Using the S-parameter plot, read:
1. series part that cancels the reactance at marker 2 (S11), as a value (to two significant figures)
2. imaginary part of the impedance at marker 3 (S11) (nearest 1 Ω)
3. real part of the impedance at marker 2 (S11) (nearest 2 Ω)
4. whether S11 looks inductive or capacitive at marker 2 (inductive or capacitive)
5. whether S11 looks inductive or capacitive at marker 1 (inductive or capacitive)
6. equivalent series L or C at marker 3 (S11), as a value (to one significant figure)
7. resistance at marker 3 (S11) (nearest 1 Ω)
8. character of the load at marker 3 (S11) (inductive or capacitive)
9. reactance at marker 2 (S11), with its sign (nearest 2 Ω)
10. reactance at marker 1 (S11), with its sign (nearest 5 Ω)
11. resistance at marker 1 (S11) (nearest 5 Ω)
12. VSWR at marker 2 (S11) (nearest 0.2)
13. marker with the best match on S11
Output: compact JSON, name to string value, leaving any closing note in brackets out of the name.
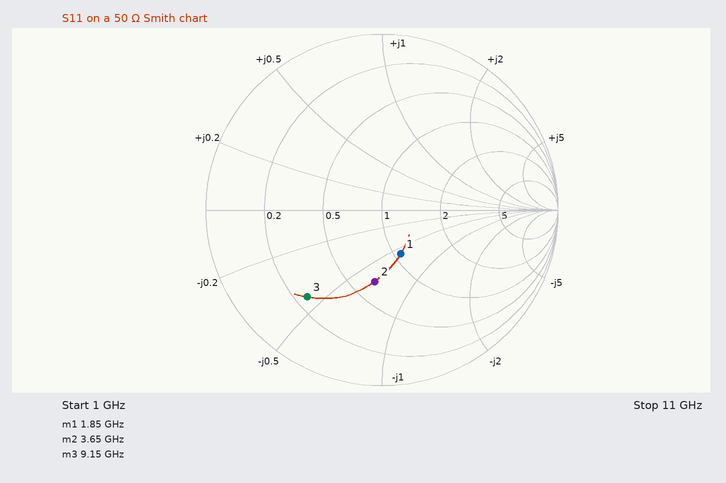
{"series part that cancels the reactance at marker 2 (S11), as a value": "1.4 nH", "imaginary part of the impedance at marker 3 (S11)": "-22 Ω", "real part of the impedance at marker 2 (S11)": "34 Ω", "whether S11 looks inductive or capacitive at marker 2": "capacitive", "whether S11 looks inductive or capacitive at marker 1": "capacitive", "equivalent series L or C at marker 3 (S11), as a value": "800 fF", "resistance at marker 3 (S11)": "13 Ω", "character of the load at marker 3 (S11)": "capacitive", "reactance at marker 2 (S11), with its sign": "-32 Ω", "reactance at marker 1 (S11), with its sign": "-30 Ω", "resistance at marker 1 (S11)": "55 Ω", "VSWR at marker 2 (S11)": "2.4", "marker with the best match on S11": "marker 1"}
